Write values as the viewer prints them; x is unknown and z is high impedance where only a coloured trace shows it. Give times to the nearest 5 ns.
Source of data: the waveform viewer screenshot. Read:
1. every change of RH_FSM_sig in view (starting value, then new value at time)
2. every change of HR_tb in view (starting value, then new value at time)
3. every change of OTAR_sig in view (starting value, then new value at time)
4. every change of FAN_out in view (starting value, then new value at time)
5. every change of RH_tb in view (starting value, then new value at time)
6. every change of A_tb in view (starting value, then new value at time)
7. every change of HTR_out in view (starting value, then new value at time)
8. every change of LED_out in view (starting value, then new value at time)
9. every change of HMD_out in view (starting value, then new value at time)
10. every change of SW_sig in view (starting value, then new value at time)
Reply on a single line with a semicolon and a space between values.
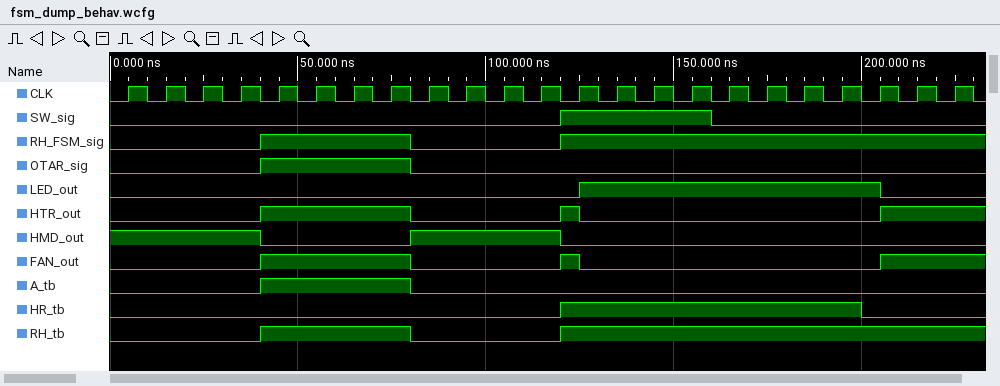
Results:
0, 1 at 40 ns, 0 at 80 ns, 1 at 120 ns; 0, 1 at 120 ns, 0 at 200 ns; 0, 1 at 40 ns, 0 at 80 ns; 0, 1 at 40 ns, 0 at 80 ns, 1 at 120 ns, 0 at 125 ns, 1 at 205 ns; 0, 1 at 40 ns, 0 at 80 ns, 1 at 120 ns; 0, 1 at 40 ns, 0 at 80 ns; 0, 1 at 40 ns, 0 at 80 ns, 1 at 120 ns, 0 at 125 ns, 1 at 205 ns; 0, 1 at 125 ns, 0 at 205 ns; 1, 0 at 40 ns, 1 at 80 ns, 0 at 120 ns; 0, 1 at 120 ns, 0 at 160 ns
